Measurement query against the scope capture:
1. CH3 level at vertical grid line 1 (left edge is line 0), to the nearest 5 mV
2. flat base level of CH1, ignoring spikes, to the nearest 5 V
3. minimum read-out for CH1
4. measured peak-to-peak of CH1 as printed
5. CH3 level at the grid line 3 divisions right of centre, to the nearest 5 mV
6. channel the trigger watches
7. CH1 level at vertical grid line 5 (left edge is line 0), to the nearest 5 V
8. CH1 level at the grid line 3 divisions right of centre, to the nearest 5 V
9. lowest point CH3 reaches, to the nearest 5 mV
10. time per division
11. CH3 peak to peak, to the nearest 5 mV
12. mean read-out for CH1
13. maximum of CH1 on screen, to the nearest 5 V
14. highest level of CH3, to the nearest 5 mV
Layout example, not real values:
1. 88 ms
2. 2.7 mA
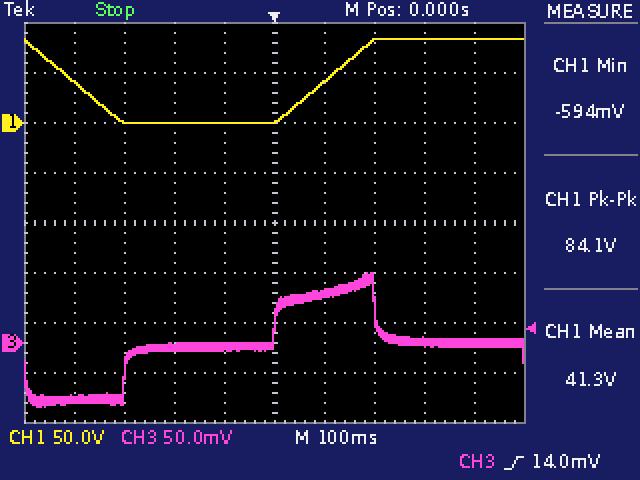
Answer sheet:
1. -55 mV
2. 0 V
3. -594 mV
4. 84.1 V
5. 0 mV
6. CH3
7. 0 V
8. 85 V
9. -65 mV
10. 100 ms
11. 135 mV
12. 41.3 V
13. 85 V
14. 70 mV
